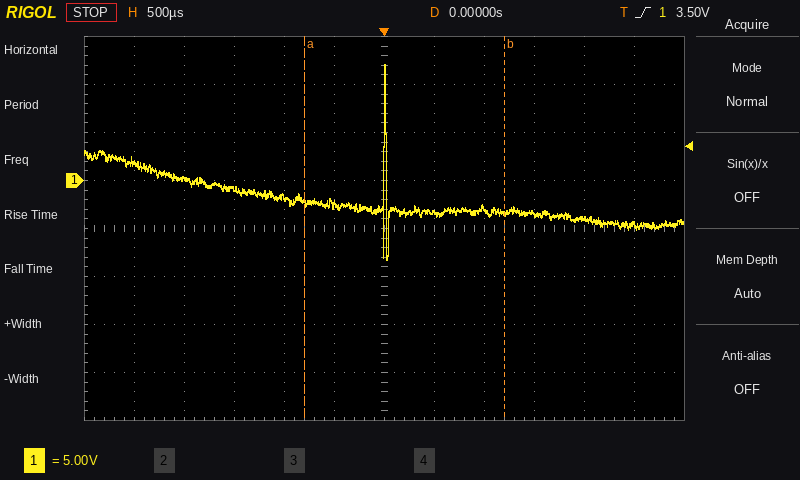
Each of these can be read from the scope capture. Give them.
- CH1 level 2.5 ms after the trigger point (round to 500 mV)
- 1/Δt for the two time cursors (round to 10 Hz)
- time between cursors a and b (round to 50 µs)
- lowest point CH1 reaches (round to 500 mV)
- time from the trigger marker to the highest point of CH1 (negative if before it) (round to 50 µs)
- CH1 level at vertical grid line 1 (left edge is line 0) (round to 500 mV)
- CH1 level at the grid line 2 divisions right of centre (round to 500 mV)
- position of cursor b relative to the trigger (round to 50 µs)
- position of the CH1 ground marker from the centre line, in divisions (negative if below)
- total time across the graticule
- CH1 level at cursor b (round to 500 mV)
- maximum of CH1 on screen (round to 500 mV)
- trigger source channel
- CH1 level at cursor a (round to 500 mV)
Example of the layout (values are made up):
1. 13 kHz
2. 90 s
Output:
1. -4.5 V
2. 500 Hz
3. 2.00 ms
4. -8.0 V
5. 0 µs
6. 2.0 V
7. -3.0 V
8. +1.20 ms
9. +1.0 div
10. 6 ms
11. -3.5 V
12. 12.0 V
13. CH1
14. -2.0 V
